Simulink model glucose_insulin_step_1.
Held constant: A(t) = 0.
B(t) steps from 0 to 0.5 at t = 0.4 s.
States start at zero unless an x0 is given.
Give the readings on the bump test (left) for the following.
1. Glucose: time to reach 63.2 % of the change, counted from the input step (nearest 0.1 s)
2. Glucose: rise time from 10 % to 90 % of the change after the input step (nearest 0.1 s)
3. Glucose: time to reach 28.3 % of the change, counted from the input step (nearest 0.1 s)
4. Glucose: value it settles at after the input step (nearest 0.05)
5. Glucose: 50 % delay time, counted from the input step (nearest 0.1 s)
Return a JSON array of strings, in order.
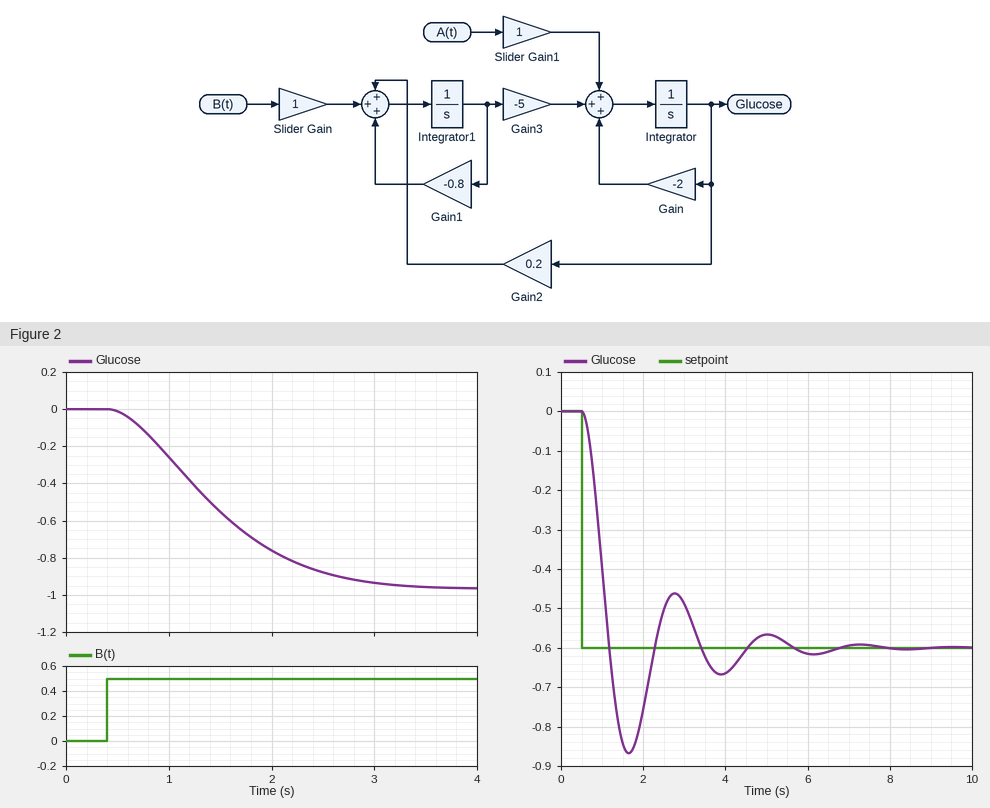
["1.2 s", "1.7 s", "0.6 s", "-0.95", "1.0 s"]
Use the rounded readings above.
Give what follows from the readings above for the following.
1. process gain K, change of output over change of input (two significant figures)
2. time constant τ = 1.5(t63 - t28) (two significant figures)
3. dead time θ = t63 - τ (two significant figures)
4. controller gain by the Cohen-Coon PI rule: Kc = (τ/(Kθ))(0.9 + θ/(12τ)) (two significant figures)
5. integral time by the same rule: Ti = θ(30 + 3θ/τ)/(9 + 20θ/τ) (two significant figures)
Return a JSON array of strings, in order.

["-1.9", "0.90 s", "0.30 s", "-1.5", "0.59 s"]
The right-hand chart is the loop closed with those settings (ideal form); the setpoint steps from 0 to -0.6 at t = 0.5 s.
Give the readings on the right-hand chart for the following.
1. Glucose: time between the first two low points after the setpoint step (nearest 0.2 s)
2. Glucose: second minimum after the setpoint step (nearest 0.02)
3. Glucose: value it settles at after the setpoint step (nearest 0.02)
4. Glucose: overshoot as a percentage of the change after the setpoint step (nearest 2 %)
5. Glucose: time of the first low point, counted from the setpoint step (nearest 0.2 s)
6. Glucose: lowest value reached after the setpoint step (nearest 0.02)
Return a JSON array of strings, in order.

["2.2 s", "-0.66", "-0.60", "44 %", "1.2 s", "-0.86"]
